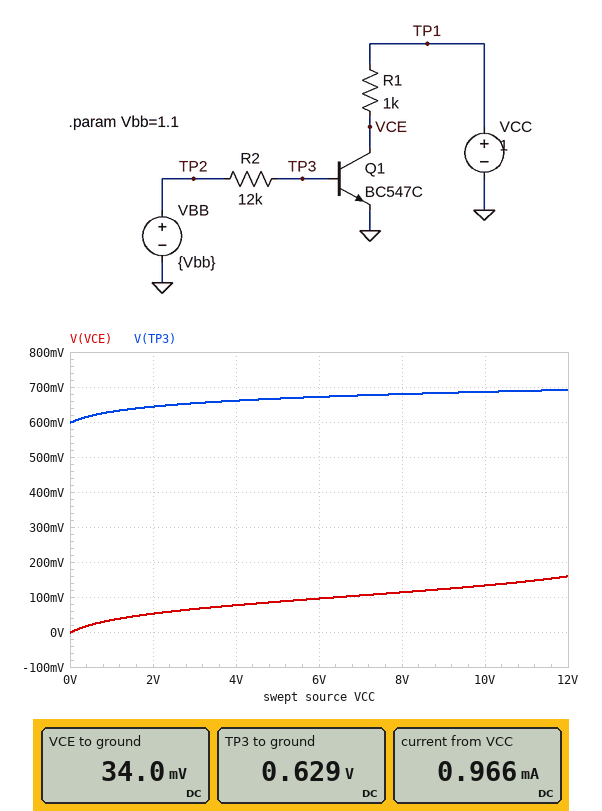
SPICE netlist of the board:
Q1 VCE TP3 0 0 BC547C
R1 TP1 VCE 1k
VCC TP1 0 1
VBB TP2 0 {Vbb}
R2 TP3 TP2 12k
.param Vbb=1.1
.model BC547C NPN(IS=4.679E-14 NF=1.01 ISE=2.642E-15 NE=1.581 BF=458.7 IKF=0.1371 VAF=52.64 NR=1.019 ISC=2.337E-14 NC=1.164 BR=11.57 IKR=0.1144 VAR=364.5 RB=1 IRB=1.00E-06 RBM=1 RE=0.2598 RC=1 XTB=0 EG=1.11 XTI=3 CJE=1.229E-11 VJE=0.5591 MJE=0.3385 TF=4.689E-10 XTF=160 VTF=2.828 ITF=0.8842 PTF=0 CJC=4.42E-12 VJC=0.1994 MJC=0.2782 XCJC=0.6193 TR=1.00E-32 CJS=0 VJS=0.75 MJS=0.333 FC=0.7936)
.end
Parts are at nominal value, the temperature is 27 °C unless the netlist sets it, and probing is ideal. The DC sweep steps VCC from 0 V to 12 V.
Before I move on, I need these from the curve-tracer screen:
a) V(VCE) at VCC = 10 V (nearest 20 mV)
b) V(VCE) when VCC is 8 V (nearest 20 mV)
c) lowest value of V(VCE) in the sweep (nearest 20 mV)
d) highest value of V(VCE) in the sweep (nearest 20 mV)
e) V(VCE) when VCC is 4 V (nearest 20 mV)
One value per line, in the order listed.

140 mV
120 mV
0 V
160 mV
80 mV
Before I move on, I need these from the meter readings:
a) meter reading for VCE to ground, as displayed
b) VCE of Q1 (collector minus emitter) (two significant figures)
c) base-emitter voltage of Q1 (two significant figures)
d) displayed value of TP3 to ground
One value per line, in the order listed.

34.0 mV
34 mV
630 mV
0.629 V
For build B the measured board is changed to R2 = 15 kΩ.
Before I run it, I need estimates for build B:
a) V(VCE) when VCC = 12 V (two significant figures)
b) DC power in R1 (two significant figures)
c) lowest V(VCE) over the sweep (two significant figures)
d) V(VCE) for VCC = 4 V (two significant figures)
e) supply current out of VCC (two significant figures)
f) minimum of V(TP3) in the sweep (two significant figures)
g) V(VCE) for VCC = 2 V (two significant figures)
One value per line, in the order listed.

530 mV
920 µW
-2.1 mV
84 mV
960 µA
590 mV
58 mV
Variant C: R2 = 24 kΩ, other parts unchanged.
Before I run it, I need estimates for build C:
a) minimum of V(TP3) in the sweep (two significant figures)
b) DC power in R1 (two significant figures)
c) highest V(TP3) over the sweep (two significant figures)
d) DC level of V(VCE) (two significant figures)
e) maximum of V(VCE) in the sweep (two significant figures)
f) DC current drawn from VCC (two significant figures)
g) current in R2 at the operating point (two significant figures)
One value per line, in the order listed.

580 mV
900 µW
680 mV
50 mV
3.9 V
950 µA
20 µA
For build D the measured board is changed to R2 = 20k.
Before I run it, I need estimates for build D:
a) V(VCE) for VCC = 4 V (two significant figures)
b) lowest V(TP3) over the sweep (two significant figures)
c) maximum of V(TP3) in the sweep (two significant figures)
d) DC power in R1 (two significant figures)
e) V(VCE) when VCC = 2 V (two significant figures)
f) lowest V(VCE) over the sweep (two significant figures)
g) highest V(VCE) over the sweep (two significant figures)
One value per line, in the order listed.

96 mV
580 mV
680 mV
910 µW
67 mV
-2.0 mV
2.7 V
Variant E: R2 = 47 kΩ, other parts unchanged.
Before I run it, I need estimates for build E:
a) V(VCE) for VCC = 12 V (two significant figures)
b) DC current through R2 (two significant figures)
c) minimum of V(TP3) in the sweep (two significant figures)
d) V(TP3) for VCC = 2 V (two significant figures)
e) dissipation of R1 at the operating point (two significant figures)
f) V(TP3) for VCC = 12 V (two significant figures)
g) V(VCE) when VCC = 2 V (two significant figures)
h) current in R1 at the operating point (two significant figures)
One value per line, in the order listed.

7.3 V
10 µA
560 mV
640 mV
870 µW
660 mV
98 mV
930 µA
